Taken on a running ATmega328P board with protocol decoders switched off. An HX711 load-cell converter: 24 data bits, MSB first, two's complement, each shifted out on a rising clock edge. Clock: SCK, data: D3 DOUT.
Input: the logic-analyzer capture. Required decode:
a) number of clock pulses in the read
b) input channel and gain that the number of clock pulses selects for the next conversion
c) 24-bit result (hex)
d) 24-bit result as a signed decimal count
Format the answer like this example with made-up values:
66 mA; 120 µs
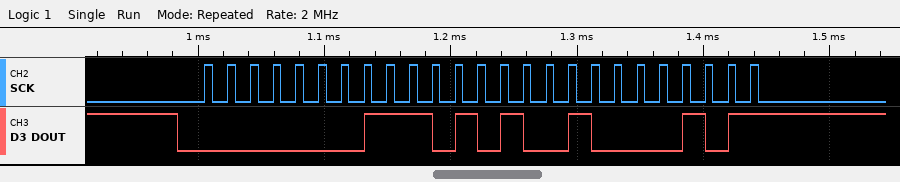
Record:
25; channel A, gain 128; 0x01D485; 119941
